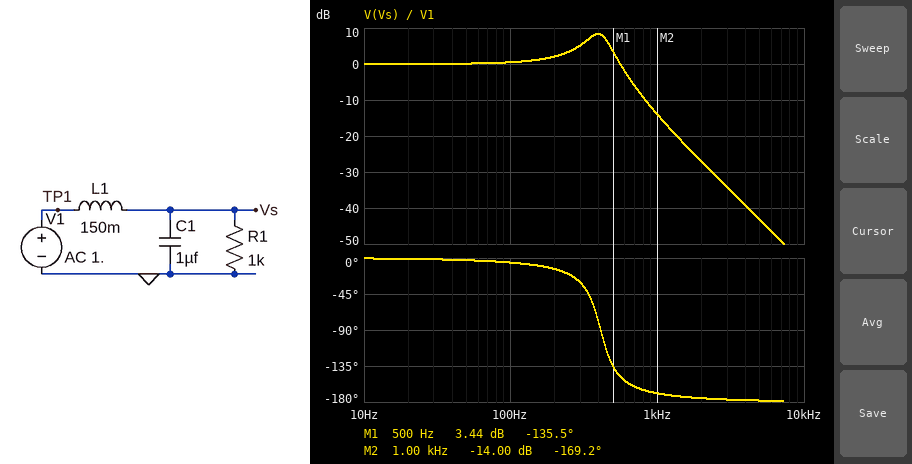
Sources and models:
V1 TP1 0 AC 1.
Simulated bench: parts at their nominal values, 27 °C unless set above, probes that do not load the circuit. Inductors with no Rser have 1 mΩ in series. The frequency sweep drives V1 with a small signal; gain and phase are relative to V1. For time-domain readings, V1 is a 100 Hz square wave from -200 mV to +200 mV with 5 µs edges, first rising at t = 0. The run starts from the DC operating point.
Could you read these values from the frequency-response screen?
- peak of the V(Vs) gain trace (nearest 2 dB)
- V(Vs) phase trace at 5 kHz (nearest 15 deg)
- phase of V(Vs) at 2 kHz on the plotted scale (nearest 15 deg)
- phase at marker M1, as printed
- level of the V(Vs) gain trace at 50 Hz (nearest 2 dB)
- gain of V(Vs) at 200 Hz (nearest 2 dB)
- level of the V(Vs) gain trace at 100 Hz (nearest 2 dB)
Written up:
8 dB
-180 deg
-180 deg
-135.5 deg
0 dB
2 dB
0 dB
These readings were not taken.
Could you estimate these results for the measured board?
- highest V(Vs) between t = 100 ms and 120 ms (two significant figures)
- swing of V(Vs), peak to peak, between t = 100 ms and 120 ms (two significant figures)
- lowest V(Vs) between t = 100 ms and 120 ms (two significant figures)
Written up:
400 mV
800 mV
-400 mV
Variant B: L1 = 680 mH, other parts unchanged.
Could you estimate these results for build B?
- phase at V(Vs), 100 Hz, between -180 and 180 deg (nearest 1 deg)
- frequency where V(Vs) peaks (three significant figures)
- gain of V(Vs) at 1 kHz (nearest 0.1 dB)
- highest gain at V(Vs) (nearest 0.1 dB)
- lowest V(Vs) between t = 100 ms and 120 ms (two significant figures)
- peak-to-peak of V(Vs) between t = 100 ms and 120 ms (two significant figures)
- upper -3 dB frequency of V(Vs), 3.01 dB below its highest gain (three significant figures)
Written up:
-30 deg
157 Hz
-28.4 dB
2.5 dB
-290 mV
590 mV
229 Hz
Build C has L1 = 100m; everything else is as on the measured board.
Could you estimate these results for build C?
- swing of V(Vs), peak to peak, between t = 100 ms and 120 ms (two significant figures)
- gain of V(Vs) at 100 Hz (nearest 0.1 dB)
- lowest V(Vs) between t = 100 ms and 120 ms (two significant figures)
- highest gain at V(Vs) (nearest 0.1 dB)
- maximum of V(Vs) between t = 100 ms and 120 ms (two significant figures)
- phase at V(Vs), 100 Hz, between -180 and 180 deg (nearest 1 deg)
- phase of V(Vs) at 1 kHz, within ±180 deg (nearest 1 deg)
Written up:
930 mV
0.3 dB
-460 mV
10.1 dB
460 mV
-4 deg
-168 deg
